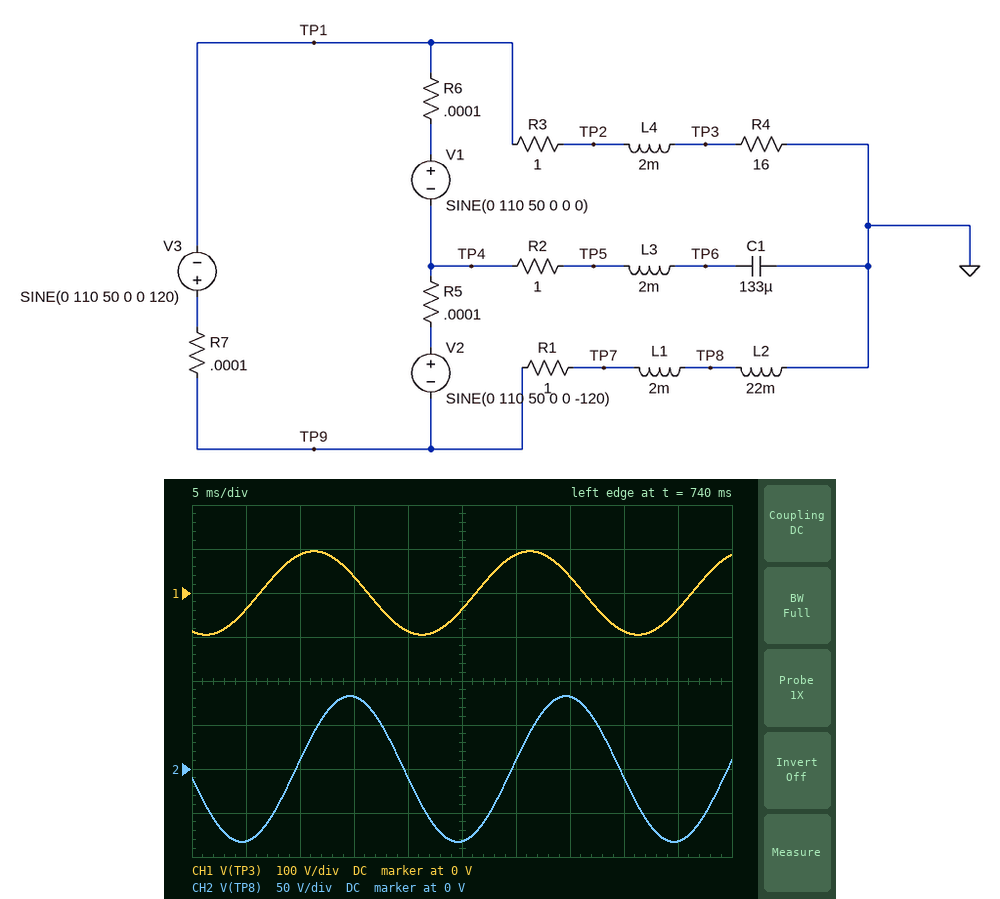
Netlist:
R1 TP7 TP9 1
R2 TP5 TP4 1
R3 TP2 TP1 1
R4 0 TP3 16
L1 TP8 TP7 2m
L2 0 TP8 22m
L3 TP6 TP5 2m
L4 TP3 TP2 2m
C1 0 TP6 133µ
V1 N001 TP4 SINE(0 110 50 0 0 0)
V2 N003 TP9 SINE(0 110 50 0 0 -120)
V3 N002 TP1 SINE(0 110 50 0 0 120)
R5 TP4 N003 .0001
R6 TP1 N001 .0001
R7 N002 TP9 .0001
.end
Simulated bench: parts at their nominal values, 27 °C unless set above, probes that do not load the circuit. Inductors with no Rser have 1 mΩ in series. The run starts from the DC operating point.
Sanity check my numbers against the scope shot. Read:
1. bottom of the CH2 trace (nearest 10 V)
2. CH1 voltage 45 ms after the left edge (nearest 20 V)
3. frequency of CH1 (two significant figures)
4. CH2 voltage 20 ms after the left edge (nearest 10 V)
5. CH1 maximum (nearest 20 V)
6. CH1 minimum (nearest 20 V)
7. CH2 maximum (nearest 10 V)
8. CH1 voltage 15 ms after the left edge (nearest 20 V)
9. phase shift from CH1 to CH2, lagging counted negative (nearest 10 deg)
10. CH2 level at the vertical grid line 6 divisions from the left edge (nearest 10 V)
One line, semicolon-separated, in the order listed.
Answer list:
-80 V; -40 V; 50 Hz; -10 V; 100 V; -100 V; 80 V; 40 V; -60 deg; 10 V
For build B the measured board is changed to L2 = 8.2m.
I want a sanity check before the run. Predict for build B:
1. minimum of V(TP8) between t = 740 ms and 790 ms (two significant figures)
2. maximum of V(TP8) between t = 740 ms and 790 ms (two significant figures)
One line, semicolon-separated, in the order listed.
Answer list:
-29 V; 29 V
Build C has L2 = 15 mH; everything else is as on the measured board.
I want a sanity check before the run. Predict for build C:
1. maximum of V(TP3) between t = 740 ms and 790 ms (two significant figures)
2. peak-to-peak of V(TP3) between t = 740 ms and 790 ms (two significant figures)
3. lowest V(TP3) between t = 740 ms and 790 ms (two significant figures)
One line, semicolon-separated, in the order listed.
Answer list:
97 V; 190 V; -97 V
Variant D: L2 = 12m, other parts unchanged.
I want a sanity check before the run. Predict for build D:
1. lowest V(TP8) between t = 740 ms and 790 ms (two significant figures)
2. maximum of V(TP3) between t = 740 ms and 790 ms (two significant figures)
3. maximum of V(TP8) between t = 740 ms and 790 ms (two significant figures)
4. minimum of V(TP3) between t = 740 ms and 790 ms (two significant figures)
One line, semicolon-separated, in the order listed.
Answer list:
-44 V; 97 V; 44 V; -97 V
